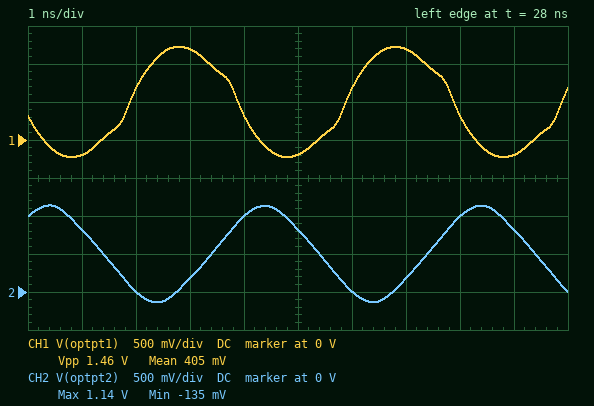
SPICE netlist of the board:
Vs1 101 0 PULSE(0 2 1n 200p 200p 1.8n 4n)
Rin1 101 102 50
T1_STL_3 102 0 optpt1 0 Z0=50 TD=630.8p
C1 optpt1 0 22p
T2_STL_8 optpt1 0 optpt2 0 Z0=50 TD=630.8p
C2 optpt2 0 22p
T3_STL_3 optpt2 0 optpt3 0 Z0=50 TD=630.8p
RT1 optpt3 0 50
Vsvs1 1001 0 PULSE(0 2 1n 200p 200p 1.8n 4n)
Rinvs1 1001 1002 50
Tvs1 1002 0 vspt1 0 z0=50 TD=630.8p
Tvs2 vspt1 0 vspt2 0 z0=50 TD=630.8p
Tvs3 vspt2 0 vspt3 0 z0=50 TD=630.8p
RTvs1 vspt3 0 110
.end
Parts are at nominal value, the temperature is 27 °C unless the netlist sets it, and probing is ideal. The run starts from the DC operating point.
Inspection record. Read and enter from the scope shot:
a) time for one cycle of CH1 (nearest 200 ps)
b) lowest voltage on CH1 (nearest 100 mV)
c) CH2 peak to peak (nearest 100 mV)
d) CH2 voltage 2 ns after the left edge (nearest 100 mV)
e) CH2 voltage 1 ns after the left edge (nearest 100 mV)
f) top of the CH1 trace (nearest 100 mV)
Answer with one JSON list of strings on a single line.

["4.0 ns", "-200 mV", "1.3 V", "0 V", "800 mV", "1.2 V"]
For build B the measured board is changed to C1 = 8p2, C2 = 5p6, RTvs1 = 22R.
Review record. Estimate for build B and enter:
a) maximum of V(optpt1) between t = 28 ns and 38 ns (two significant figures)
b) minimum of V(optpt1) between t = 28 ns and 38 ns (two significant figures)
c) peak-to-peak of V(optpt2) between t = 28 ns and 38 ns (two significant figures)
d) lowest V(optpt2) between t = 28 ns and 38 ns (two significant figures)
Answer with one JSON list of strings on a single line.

["1.0 V", "-24 mV", "1.2 V", "-110 mV"]
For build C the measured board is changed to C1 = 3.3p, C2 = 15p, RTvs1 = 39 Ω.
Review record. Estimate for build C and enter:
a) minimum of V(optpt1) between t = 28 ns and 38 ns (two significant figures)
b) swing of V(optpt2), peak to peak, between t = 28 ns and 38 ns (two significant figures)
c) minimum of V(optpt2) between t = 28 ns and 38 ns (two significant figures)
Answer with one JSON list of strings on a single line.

["-190 mV", "1.1 V", "-64 mV"]
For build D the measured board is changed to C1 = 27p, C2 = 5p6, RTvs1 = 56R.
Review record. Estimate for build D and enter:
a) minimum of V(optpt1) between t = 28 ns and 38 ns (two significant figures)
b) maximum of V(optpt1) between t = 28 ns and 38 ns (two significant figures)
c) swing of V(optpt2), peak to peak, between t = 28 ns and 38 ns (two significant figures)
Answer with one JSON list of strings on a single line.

["110 mV", "890 mV", "1.0 V"]
